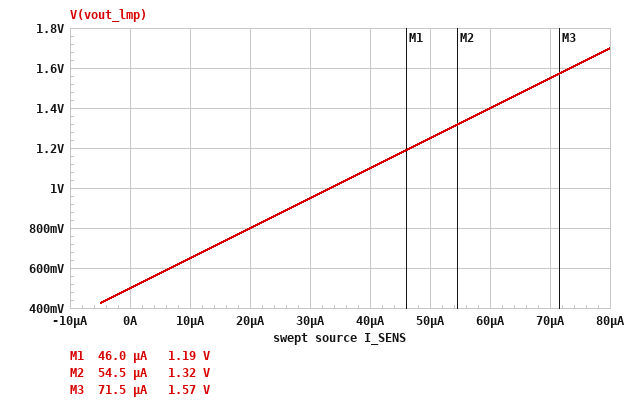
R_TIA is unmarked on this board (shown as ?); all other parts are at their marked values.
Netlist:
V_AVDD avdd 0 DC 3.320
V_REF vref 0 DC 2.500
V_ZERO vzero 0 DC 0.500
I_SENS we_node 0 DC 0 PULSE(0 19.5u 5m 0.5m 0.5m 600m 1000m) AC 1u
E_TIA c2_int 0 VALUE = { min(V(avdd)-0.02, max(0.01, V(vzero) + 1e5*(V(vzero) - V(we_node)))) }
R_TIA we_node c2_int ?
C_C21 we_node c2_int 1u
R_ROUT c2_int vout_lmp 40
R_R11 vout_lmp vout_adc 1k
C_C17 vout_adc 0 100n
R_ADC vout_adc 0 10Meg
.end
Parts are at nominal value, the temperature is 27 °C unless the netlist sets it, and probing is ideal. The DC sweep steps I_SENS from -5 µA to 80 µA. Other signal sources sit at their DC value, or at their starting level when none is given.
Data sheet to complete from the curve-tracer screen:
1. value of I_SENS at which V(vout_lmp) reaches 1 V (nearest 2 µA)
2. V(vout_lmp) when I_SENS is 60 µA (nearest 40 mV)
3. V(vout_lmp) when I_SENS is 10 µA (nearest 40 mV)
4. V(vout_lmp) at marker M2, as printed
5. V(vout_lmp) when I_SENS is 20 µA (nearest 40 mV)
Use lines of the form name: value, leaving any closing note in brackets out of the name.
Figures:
value of I_SENS at which V(vout_lmp) reaches 1 V: 34 µA
V(vout_lmp) when I_SENS is 60 µA: 1.40 V
V(vout_lmp) when I_SENS is 10 µA: 640 mV
V(vout_lmp) at marker M2, as printed: 1.32 V
V(vout_lmp) when I_SENS is 20 µA: 800 mV
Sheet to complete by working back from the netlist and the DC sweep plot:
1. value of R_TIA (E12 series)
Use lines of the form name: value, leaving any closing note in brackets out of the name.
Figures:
value of R_TIA: 15 kΩ
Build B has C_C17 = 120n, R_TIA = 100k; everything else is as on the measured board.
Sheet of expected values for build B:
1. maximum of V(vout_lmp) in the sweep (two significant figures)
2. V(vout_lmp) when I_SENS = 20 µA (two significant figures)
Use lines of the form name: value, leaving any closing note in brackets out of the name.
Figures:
maximum of V(vout_lmp) in the sweep: 3.3 V
V(vout_lmp) when I_SENS = 20 µA: 2.5 V
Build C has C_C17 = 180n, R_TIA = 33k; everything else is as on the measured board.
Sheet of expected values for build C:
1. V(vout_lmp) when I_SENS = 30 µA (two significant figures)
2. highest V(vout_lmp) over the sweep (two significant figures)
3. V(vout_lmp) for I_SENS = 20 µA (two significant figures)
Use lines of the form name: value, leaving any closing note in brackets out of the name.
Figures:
V(vout_lmp) when I_SENS = 30 µA: 1.5 V
highest V(vout_lmp) over the sweep: 3.1 V
V(vout_lmp) for I_SENS = 20 µA: 1.2 V
